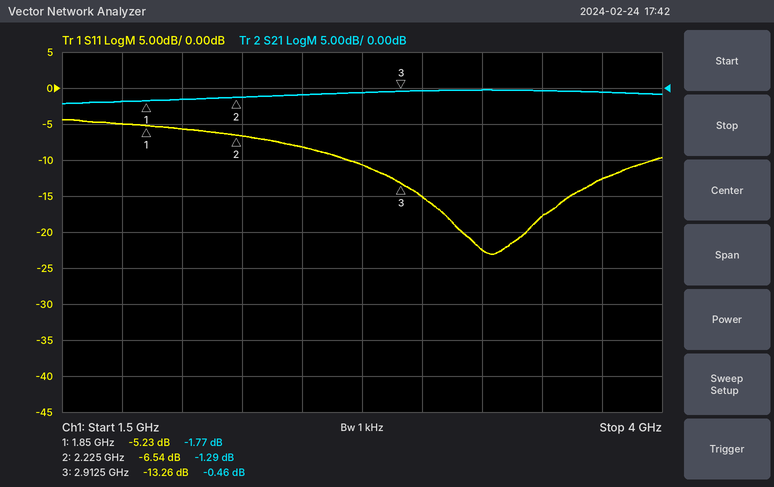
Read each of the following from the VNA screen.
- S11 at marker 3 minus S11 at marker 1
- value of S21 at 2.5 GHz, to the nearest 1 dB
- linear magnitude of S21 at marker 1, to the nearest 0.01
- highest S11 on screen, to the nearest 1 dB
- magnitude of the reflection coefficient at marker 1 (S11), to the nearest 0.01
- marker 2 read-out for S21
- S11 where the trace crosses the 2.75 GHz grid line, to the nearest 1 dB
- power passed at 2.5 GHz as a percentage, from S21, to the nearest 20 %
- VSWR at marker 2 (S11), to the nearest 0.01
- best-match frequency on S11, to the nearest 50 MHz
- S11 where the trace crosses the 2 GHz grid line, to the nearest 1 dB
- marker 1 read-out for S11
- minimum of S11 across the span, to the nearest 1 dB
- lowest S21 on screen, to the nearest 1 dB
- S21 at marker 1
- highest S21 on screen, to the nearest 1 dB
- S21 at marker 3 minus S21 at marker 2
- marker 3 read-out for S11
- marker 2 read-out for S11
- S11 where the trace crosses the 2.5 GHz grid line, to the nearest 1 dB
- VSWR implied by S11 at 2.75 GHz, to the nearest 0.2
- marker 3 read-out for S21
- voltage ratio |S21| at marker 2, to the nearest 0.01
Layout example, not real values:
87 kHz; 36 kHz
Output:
-8.03 dB; -1 dB; 0.82; -4 dB; 0.55; -1.29 dB; -11 dB; 80 %; 2.78; 3.30 GHz; -6 dB; -5.23 dB; -23 dB; -2 dB; -1.77 dB; 0 dB; 0.83 dB; -13.26 dB; -6.54 dB; -8 dB; 1.8; -0.46 dB; 0.86
